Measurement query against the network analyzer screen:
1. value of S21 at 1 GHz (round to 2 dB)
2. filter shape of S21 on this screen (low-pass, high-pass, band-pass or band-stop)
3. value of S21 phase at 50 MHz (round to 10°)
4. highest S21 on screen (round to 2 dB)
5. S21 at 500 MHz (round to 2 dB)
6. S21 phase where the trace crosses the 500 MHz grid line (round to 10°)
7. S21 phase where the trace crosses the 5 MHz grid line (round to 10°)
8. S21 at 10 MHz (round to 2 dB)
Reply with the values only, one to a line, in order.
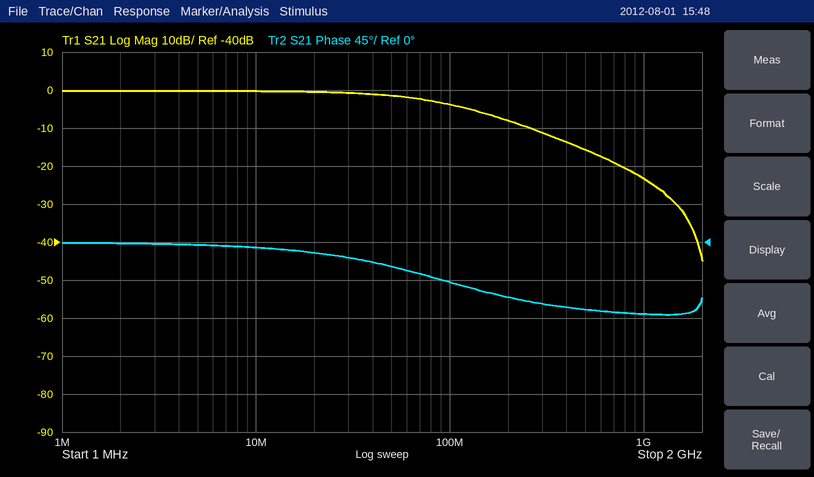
-24 dB
low-pass
-30°
0 dB
-16 dB
-80°
0°
0 dB
